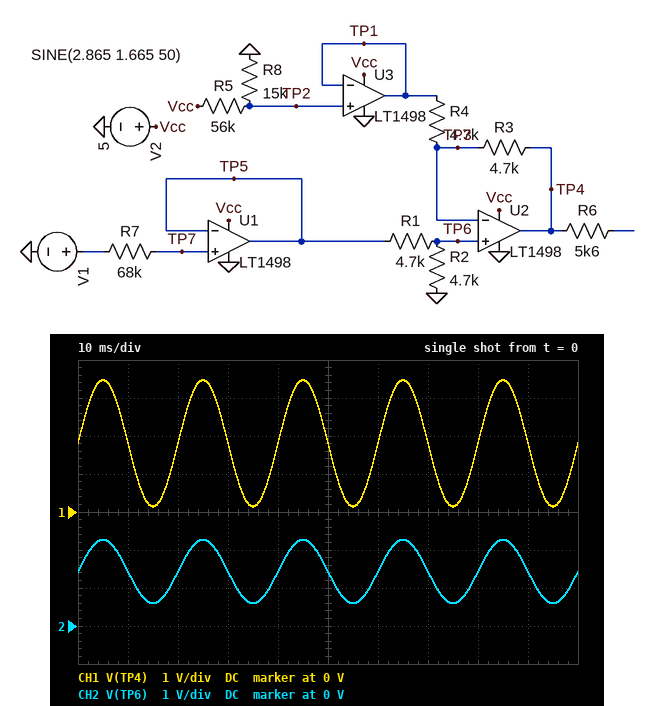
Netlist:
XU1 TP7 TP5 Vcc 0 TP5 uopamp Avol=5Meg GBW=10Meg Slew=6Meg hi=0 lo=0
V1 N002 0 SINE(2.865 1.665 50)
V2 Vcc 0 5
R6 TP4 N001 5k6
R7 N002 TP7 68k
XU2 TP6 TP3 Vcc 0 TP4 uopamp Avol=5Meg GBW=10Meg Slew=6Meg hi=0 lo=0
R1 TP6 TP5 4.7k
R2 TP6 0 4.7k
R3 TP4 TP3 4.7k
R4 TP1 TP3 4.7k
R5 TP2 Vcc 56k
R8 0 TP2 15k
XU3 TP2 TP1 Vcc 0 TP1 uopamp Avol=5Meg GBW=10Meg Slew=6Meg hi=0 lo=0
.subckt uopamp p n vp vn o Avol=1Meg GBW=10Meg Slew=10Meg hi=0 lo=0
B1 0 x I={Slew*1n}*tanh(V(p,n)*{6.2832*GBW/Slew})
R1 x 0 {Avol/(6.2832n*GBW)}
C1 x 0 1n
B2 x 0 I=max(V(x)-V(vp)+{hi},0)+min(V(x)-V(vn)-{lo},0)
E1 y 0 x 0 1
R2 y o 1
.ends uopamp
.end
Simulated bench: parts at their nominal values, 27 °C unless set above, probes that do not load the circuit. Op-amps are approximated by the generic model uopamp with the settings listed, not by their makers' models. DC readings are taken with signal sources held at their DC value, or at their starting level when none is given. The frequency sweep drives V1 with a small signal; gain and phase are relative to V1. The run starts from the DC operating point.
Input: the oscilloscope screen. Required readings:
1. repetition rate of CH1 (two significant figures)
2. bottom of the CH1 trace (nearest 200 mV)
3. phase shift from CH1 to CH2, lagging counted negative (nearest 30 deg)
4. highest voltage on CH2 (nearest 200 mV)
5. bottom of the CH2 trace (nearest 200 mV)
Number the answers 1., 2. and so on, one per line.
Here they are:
1. 50 Hz
2. 200 mV
3. 0 deg
4. 2.2 V
5. 600 mV
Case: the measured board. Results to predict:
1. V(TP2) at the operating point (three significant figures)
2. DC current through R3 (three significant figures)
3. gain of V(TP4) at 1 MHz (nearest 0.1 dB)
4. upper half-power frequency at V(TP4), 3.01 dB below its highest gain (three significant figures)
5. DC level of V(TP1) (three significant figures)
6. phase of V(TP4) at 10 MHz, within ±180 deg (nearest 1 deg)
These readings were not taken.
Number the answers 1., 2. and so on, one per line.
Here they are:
1. 1.06 V
2. 80.0 µA
3. -0.2 dB
4. 4.19 MHz
5. 1.06 V
6. -108 deg
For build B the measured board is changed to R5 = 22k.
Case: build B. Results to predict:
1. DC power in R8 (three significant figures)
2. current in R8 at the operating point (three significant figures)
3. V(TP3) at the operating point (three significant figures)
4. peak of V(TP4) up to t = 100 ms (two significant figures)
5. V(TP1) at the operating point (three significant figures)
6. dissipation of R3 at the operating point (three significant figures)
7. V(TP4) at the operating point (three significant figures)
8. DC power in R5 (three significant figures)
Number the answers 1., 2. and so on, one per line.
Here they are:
1. 274 µW
2. 135 µA
3. 1.43 V
4. 2.5 V
5. 2.03 V
6. 75.2 µW
7. 838 mV
8. 402 µW
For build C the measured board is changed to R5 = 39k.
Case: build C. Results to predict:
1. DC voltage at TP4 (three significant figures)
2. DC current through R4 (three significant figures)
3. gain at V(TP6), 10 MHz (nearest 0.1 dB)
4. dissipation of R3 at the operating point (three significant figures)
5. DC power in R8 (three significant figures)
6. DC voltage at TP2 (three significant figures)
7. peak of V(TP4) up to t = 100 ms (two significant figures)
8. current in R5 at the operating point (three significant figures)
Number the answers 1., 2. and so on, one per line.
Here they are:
1. 1.48 V
2. 9.28 µA
3. -9.0 dB
4. 405 nW
5. 129 µW
6. 1.39 V
7. 3.1 V
8. 92.6 µA
